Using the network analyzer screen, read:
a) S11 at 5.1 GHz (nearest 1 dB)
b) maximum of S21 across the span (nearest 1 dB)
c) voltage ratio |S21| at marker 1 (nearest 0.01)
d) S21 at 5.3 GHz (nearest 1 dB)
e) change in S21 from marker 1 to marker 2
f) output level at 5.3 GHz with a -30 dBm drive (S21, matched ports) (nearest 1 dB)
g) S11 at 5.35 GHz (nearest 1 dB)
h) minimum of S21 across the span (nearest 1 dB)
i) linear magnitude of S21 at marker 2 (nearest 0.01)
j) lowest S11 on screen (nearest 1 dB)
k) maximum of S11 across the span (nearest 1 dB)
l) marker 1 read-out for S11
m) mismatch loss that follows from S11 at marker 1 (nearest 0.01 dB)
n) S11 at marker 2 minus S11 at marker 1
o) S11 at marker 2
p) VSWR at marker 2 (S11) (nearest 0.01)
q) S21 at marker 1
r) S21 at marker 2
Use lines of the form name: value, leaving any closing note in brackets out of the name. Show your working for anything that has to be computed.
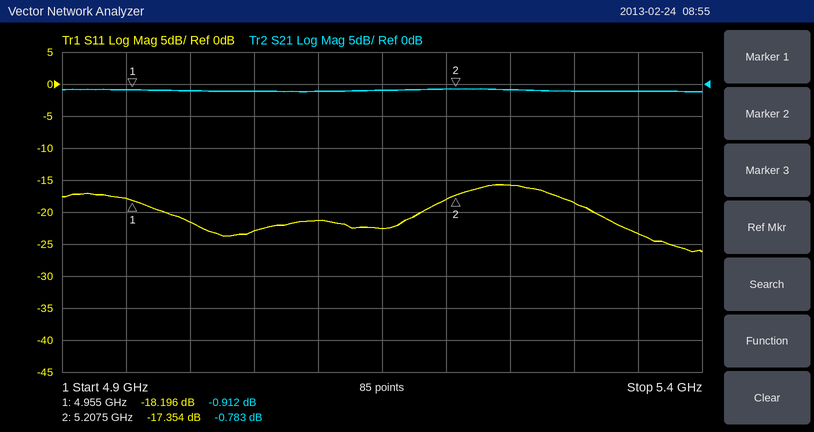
S11 at 5.1 GHz: -21 dB
maximum of S21 across the span: -1 dB
voltage ratio |S21| at marker 1: 10^(-0.912/20) ≈ 0.90
S21 at 5.3 GHz: -1 dB
change in S21 from marker 1 to marker 2: -0.783 − (-0.912) = 0.129 dB
output level at 5.3 GHz with a -30 dBm drive (S21, matched ports): -30 dBm + (-1 dB) = -31 dBm
S11 at 5.35 GHz: -23 dB
minimum of S21 across the span: -1 dB
linear magnitude of S21 at marker 2: 10^(-0.783/20) ≈ 0.91
lowest S11 on screen: -26 dB
maximum of S11 across the span: -16 dB
marker 1 read-out for S11: -18.196 dB
mismatch loss that follows from S11 at marker 1: −10 log10(1 − 10^(-18.196/10)) ≈ 0.07 dB
S11 at marker 2 minus S11 at marker 1: -17.354 − (-18.196) = 0.842 dB
S11 at marker 2: -17.354 dB
VSWR at marker 2 (S11): (1 + 0.1356)/(1 − 0.1356) ≈ 1.31
S21 at marker 1: -0.912 dB
S21 at marker 2: -0.783 dB
